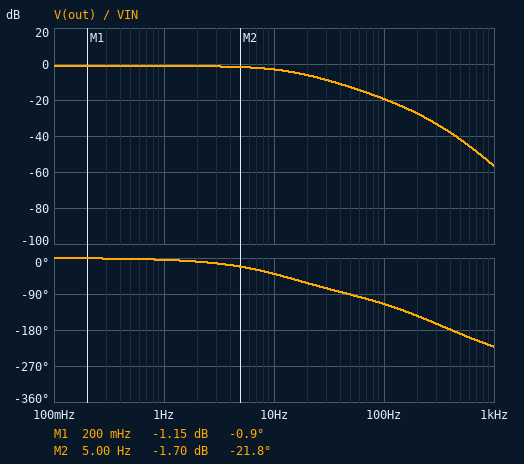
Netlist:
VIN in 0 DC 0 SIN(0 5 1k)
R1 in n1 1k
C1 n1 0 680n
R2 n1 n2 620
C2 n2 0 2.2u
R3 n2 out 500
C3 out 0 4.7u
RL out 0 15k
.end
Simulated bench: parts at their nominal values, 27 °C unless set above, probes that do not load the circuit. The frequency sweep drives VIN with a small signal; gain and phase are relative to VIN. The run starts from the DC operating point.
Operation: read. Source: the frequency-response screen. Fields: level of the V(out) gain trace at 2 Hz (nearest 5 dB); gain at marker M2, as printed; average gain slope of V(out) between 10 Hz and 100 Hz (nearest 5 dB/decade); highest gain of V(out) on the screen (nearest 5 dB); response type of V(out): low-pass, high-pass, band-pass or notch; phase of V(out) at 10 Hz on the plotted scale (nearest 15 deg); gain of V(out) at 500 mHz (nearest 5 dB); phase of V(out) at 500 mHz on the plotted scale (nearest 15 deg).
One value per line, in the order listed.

0 dB
-1.70 dB
-15 dB/decade
0 dB
low-pass
-45 deg
0 dB
0 deg
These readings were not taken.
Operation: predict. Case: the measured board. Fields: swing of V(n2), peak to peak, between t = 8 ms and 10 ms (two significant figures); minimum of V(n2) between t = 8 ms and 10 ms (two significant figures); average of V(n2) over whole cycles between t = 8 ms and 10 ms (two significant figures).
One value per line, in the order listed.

220 mV
-84 mV
26 mV
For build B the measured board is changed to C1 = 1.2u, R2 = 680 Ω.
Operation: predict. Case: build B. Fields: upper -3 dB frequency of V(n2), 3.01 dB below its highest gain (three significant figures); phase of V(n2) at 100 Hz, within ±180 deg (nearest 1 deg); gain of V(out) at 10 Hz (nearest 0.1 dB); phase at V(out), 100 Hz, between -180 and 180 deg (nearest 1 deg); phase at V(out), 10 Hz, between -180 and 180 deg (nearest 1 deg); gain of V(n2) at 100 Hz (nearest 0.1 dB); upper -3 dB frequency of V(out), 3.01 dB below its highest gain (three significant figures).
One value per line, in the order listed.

13.4 Hz
-68 deg
-3.2 dB
-123 deg
-42 deg
-15.1 dB
13.0 Hz
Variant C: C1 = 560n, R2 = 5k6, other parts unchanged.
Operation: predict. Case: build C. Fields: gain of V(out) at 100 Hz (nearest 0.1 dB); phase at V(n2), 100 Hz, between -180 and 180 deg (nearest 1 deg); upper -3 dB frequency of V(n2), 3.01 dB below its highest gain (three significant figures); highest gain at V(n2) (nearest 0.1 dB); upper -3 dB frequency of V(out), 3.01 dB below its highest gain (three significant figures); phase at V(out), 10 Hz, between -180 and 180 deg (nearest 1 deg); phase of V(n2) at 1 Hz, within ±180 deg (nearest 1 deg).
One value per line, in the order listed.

-30.7 dB
-73 deg
4.97 Hz
-3.1 dB
4.94 Hz
-68 deg
-11 deg
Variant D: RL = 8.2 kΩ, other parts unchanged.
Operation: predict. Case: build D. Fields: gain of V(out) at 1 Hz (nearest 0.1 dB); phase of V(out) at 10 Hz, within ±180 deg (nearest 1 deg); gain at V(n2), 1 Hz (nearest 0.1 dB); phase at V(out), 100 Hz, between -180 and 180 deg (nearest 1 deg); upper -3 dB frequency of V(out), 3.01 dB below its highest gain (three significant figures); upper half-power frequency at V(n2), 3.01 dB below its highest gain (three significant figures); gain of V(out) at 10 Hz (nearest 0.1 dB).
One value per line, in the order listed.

-2.0 dB
-37 deg
-1.5 dB
-114 deg
15.0 Hz
15.7 Hz
-3.6 dB
